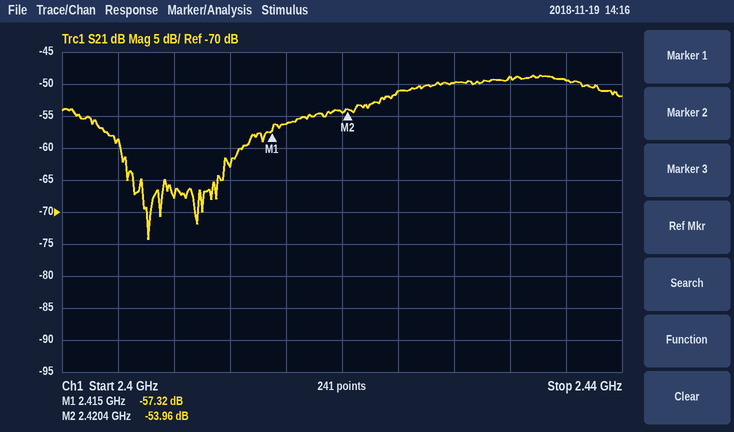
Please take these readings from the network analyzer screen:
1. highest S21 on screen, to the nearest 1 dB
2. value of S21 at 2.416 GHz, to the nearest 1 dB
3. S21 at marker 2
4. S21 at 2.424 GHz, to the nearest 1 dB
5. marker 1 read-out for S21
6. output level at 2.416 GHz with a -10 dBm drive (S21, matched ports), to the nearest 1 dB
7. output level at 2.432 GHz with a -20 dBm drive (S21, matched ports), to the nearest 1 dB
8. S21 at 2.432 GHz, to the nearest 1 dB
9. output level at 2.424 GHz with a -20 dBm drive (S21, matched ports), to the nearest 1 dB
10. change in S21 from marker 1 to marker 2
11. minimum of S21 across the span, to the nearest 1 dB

-49 dB
-56 dB
-53.96 dB
-51 dB
-57.32 dB
-66 dBm
-69 dBm
-49 dB
-71 dBm
3.36 dB
-74 dB
